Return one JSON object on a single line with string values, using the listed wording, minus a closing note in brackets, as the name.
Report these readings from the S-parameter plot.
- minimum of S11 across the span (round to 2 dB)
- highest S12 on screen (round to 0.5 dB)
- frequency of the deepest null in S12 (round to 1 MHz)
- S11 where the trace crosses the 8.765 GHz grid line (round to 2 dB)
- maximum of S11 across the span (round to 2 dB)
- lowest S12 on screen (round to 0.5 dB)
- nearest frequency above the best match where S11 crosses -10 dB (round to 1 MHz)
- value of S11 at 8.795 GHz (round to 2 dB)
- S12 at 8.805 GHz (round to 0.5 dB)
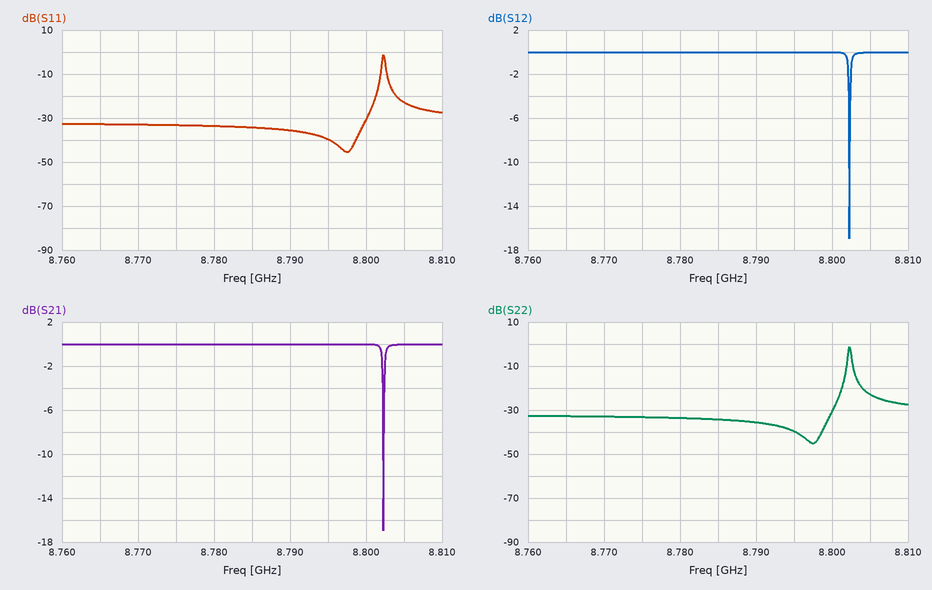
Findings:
{"minimum of S11 across the span": "-46 dB", "highest S12 on screen": "0.0 dB", "frequency of the deepest null in S12": "8.802 GHz", "S11 where the trace crosses the 8.765 GHz grid line": "-32 dB", "maximum of S11 across the span": "-2 dB", "lowest S12 on screen": "-17.0 dB", "nearest frequency above the best match where S11 crosses -10 dB": "8.802 GHz", "value of S11 at 8.795 GHz": "-40 dB", "S12 at 8.805 GHz": "0.0 dB"}
